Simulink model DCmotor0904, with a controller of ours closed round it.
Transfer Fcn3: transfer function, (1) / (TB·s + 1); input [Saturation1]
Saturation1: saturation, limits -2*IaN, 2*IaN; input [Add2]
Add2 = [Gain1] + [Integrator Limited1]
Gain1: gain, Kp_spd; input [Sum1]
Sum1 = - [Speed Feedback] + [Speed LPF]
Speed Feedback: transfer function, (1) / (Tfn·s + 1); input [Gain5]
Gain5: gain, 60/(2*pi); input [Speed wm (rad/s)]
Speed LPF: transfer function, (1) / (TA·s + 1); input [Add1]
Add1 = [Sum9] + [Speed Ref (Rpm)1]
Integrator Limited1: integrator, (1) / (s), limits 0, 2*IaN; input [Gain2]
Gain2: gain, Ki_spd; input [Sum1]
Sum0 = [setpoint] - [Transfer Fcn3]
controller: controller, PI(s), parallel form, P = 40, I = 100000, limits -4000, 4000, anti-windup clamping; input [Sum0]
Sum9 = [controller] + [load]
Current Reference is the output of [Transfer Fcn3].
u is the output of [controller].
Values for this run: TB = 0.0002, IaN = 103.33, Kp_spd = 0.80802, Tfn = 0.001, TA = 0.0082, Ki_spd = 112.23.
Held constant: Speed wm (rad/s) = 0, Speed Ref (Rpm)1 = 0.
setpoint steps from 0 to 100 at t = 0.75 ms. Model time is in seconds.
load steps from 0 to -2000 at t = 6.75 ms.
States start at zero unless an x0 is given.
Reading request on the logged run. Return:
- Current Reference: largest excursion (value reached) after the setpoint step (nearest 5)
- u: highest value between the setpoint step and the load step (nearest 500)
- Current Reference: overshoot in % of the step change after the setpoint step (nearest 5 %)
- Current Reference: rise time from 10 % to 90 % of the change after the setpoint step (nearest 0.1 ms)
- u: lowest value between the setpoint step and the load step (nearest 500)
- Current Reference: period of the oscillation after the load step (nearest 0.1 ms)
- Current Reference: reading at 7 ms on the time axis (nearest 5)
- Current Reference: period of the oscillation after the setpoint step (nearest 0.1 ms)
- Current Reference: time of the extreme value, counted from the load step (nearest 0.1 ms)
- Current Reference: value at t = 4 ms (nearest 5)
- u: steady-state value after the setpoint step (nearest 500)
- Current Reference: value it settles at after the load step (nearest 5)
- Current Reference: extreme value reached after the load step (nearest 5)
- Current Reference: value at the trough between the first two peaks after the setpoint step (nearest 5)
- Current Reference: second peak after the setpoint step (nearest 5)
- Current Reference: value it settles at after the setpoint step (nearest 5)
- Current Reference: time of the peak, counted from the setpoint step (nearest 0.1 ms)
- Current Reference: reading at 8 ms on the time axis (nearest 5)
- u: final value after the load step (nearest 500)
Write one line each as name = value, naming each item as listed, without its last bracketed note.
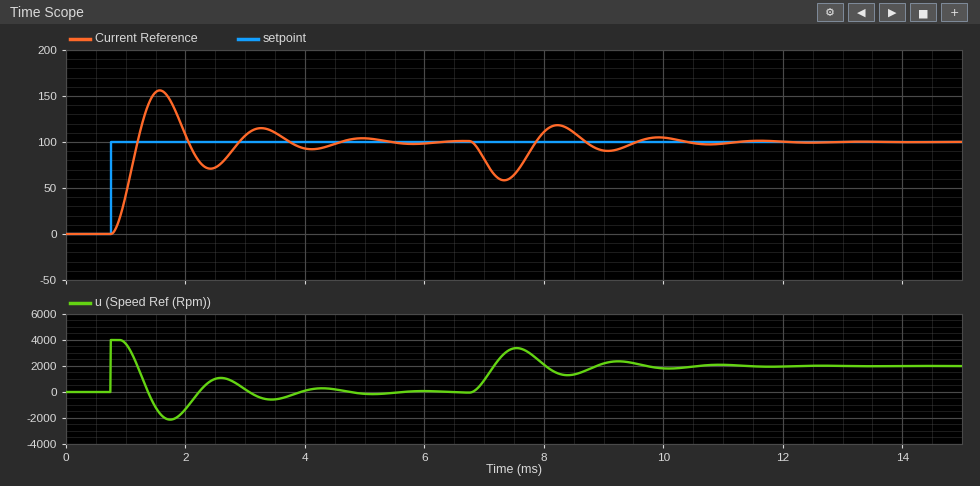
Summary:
Current Reference: largest excursion (value reached) after the setpoint step = 155
u: highest value between the setpoint step and the load step = 4000
Current Reference: overshoot in % of the step change after the setpoint step = 55 %
Current Reference: rise time from 10 % to 90 % of the change after the setpoint step = 0.3 ms
u: lowest value between the setpoint step and the load step = -2000
Current Reference: period of the oscillation after the load step = 1.7 ms
Current Reference: reading at 7 ms on the time axis = 80
Current Reference: period of the oscillation after the setpoint step = 1.7 ms
Current Reference: time of the extreme value, counted from the load step = 0.6 ms
Current Reference: value at t = 4 ms = 95
u: steady-state value after the setpoint step = 0
Current Reference: value it settles at after the load step = 100
Current Reference: extreme value reached after the load step = 60
Current Reference: value at the trough between the first two peaks after the setpoint step = 70
Current Reference: second peak after the setpoint step = 115
Current Reference: value it settles at after the setpoint step = 100
Current Reference: time of the peak, counted from the setpoint step = 0.8 ms
Current Reference: reading at 8 ms on the time axis = 110
u: final value after the load step = 2000
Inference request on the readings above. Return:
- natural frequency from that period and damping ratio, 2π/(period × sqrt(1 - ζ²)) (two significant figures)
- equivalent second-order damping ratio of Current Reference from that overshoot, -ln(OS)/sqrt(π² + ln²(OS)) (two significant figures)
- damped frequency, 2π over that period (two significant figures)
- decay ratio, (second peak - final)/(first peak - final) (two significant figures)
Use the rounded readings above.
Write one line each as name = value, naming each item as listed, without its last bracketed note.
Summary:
natural frequency from that period and damping ratio, 2π/(period × sqrt(1 - ζ²)) = 3.8 rad/ms
equivalent second-order damping ratio of Current Reference from that overshoot, -ln(OS)/sqrt(π² + ln²(OS)) = 0.19
damped frequency, 2π over that period = 3.7 rad/ms
decay ratio, (second peak - final)/(first peak - final) = 0.27
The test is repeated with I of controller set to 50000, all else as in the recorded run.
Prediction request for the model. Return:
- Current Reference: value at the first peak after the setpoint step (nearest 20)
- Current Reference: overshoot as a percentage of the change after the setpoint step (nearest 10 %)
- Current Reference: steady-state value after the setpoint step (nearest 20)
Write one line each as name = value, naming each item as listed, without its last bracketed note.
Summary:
Current Reference: value at the first peak after the setpoint step = 140
Current Reference: overshoot as a percentage of the change after the setpoint step = 40 %
Current Reference: steady-state value after the setpoint step = 100
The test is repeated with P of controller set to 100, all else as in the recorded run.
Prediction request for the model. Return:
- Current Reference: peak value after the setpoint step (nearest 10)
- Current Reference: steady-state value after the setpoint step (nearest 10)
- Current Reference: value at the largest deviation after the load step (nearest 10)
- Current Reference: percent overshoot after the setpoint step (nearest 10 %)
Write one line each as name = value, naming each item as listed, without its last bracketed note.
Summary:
Current Reference: peak value after the setpoint step = 120
Current Reference: steady-state value after the setpoint step = 100
Current Reference: value at the largest deviation after the load step = 80
Current Reference: percent overshoot after the setpoint step = 20 %
